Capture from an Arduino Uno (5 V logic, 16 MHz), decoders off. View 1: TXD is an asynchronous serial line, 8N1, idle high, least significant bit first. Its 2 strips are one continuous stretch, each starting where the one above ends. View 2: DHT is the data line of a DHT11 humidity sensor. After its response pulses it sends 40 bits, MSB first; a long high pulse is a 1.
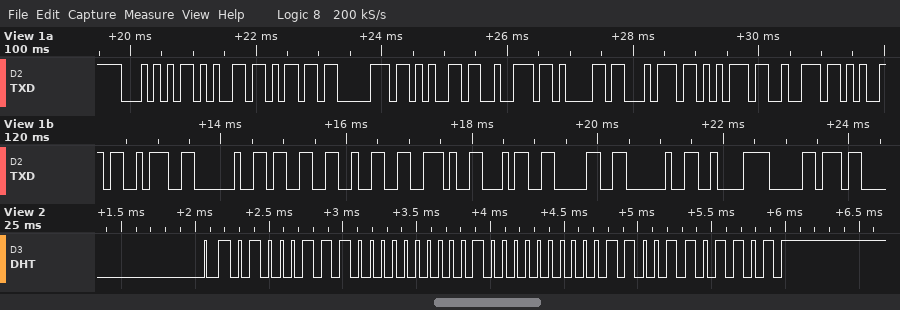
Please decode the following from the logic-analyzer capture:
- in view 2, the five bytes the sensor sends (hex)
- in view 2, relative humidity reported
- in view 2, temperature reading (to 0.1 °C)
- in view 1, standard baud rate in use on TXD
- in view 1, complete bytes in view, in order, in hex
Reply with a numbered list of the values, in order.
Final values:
1. 47 00 20 06 6D
2. 71 %
3. 32.6 °C
4. 9600 baud
5. 54 65 6D 70 65 72 61 74 75 72 65 3A 20 33 32 2E 34 30 20 C2 B0
